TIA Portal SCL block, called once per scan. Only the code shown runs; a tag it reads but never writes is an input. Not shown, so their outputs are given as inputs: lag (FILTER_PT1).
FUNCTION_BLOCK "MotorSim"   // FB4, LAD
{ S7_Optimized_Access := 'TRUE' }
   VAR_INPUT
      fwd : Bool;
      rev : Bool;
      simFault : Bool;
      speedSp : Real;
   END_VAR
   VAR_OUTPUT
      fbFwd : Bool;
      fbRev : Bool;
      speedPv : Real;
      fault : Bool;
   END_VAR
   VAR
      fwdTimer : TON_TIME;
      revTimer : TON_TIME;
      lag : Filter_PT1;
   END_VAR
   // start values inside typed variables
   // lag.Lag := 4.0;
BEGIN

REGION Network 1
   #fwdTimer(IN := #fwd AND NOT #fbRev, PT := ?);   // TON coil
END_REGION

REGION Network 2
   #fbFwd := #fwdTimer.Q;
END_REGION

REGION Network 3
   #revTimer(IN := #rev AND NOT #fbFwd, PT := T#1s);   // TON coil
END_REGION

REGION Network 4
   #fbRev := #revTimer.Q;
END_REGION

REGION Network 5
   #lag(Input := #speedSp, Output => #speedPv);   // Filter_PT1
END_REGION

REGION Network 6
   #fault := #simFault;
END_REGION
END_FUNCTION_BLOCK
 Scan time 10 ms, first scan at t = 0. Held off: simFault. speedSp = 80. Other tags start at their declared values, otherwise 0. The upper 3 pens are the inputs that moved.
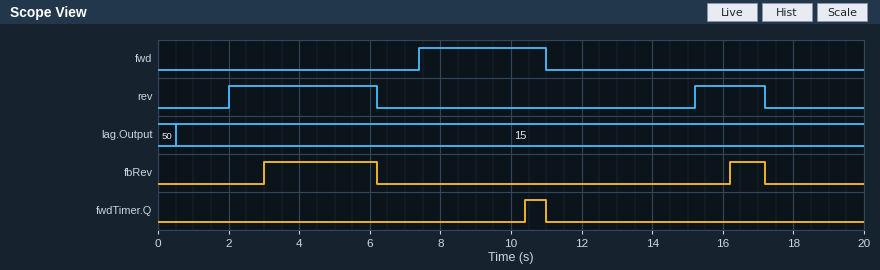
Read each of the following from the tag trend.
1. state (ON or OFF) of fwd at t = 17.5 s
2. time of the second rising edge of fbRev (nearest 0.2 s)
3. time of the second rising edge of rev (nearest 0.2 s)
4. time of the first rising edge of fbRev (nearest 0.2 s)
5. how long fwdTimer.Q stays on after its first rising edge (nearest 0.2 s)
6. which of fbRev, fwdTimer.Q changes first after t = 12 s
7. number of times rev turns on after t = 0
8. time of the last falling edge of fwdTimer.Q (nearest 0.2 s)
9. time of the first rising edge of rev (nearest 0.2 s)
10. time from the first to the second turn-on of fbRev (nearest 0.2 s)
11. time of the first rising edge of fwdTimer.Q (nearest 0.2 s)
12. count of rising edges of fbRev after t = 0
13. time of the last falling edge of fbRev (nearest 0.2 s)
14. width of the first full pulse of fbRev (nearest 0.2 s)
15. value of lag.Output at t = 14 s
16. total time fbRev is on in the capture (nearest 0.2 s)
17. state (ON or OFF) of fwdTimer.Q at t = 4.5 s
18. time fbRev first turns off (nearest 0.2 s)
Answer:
OFF
16.2 s
15.2 s
3.0 s
0.6 s
fbRev
2
11.0 s
2.0 s
13.2 s
10.4 s
2
17.2 s
3.2 s
15
4.2 s
OFF
6.2 s
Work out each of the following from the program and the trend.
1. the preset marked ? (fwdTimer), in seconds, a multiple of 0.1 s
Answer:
3.0 s
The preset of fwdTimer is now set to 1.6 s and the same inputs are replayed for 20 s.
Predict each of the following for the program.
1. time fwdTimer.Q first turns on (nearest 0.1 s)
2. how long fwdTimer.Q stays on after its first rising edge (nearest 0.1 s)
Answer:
9.0 s
2.0 s
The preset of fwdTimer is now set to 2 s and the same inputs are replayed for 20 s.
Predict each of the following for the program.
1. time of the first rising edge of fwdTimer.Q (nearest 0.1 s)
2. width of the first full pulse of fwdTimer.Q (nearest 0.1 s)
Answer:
9.4 s
1.6 s
